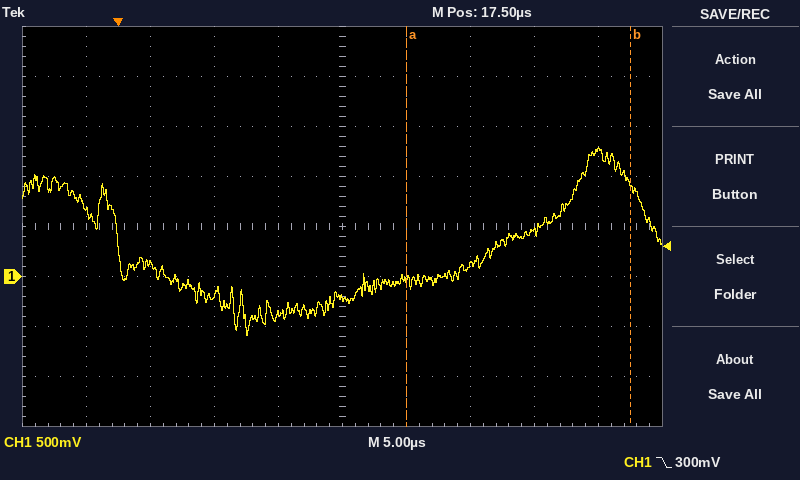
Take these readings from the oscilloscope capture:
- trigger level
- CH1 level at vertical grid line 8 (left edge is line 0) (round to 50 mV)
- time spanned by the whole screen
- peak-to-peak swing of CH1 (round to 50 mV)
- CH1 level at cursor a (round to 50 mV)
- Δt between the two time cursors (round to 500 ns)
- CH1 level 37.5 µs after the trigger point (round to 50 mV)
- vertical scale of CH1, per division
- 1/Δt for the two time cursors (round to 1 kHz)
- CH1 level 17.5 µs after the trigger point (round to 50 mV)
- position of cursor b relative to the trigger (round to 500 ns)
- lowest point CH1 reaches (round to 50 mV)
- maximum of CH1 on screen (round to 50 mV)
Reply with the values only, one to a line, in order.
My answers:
300 mV
450 mV
50 µs
1.90 V
-50 mV
17.5 µs
1.25 V
500 mV
57 kHz
-200 mV
+40.0 µs
-600 mV
1.30 V
